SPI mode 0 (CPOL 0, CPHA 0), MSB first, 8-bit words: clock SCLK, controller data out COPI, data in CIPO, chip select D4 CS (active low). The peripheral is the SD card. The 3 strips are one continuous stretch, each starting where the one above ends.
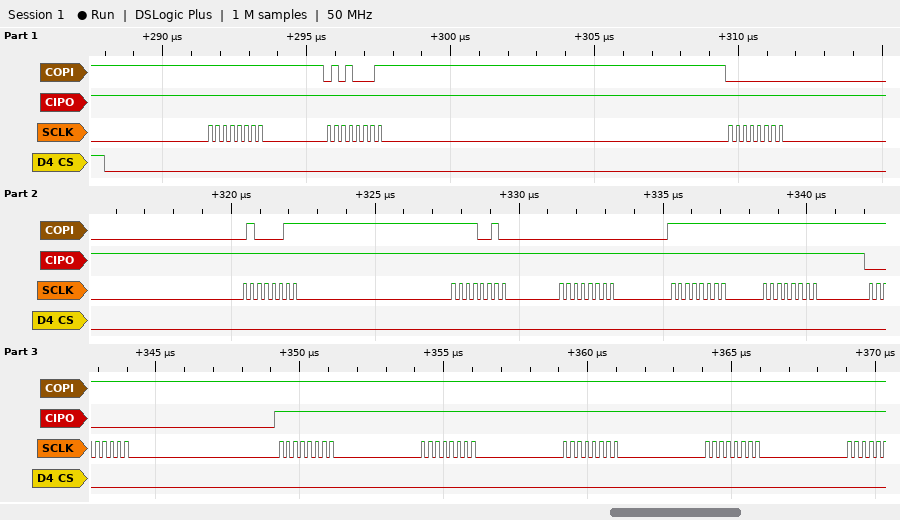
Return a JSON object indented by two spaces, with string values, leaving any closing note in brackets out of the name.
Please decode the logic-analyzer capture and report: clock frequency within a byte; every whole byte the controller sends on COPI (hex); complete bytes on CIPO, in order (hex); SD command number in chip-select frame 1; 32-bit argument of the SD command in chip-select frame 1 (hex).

{
  "clock frequency within a byte": "4 MHz",
  "every whole byte the controller sends on COPI": "0xFF 0x51 0x00 0x43 0xF2 0x00 0xFF 0xFF 0xFF 0xFF 0xFF 0xFF 0xFF",
  "complete bytes on CIPO, in order": "0xFF 0xFF 0xFF 0xFF 0xFF 0xFF 0xFF 0xFF 0x00 0xFF 0xFF 0xFF 0xFF",
  "SD command number in chip-select frame 1": "CMD17",
  "32-bit argument of the SD command in chip-select frame 1": "0x0043F200"
}
